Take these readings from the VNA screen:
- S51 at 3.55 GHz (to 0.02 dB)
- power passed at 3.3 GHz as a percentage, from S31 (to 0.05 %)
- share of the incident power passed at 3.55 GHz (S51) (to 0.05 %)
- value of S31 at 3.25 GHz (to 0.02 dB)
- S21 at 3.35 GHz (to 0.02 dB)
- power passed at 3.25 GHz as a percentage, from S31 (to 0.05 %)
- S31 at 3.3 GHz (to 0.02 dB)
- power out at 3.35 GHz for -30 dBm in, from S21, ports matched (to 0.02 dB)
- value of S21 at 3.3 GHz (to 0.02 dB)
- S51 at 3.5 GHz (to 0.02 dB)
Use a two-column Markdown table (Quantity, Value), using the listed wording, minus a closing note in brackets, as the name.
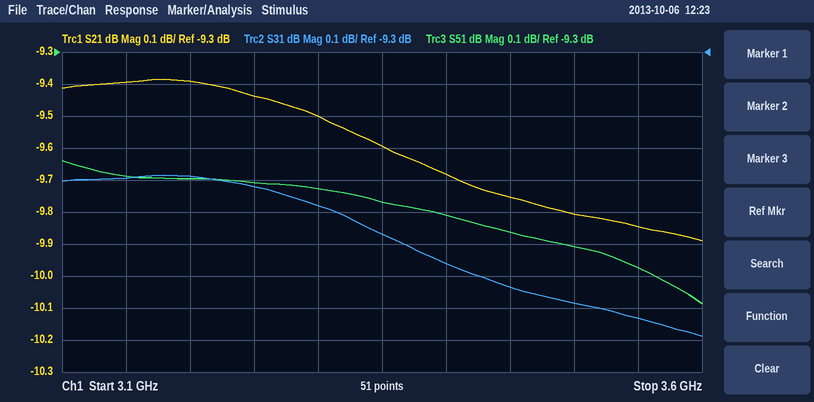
| Quantity | Value |
|---|---|
| S51 at 3.55 GHz | -9.98 dB |
| power passed at 3.3 GHz as a percentage, from S31 | 10.50 % |
| share of the incident power passed at 3.55 GHz (S51) | 10.05 % |
| value of S31 at 3.25 GHz | -9.72 dB |
| S21 at 3.35 GHz | -9.60 dB |
| power passed at 3.25 GHz as a percentage, from S31 | 10.65 % |
| S31 at 3.3 GHz | -9.78 dB |
| power out at 3.35 GHz for -30 dBm in, from S21, ports matched | -39.60 dBm |
| value of S21 at 3.3 GHz | -9.50 dB |
| S51 at 3.5 GHz | -9.90 dB |
